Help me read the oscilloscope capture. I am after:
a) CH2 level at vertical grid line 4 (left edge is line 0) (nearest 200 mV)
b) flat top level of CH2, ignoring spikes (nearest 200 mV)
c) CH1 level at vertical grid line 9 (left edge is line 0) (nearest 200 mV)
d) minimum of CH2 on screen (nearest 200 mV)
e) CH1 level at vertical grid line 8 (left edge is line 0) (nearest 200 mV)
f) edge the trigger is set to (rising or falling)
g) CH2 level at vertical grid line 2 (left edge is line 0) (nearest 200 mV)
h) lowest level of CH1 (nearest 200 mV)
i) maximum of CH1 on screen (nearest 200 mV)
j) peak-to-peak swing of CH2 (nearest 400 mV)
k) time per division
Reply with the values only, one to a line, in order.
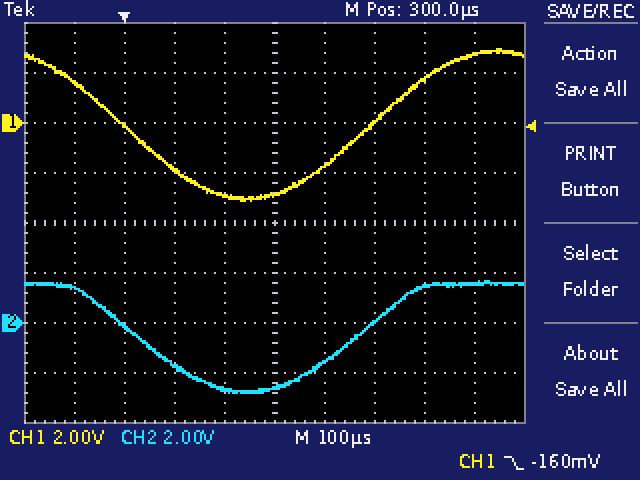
-2.6 V
1.6 V
2.8 V
-2.8 V
1.8 V
falling
-200 mV
-3.2 V
3.0 V
4.4 V
100 µs
